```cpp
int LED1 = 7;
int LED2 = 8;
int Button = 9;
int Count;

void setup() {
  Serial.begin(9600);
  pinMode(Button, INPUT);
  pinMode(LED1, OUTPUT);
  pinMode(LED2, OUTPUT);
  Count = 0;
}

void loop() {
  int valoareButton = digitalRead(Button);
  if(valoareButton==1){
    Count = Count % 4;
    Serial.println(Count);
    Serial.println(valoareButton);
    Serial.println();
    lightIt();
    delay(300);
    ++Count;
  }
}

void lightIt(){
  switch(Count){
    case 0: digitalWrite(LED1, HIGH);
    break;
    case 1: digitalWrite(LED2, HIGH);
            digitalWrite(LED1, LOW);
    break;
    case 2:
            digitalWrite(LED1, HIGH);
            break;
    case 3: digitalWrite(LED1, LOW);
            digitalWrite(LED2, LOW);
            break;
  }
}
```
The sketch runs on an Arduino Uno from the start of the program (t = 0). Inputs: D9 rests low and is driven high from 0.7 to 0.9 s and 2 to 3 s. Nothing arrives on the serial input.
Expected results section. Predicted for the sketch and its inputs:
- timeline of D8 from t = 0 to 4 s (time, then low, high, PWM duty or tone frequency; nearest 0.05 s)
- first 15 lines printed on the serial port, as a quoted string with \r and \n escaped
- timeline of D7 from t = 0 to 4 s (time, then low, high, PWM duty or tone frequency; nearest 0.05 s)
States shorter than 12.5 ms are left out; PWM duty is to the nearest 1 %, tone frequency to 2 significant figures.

0 s low; 2 s high; 2.6 s low
"0\r\n1\r\n\r\n1\r\n1\r\n\r\n2\r\n1\r\n\r\n3\r\n1\r\n\r\n0\r\n1\r\n\r\n"
0 s low; 0.7 s high; 2 s low; 2.3 s high; 2.6 s low; 2.9 s high
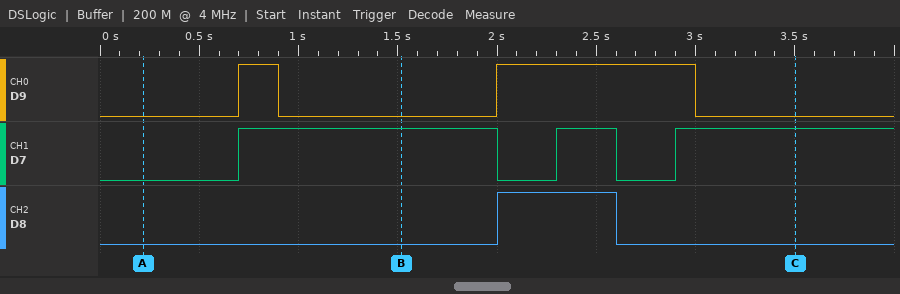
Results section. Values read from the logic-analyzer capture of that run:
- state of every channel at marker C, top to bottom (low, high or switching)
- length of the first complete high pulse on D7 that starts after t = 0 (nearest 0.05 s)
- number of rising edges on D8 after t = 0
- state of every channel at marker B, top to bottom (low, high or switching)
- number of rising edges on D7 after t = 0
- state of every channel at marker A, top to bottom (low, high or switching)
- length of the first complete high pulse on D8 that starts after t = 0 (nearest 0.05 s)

D9 low, D7 high, D8 low
1.30 s
1
D9 low, D7 high, D8 low
3
D9 low, D7 low, D8 low
0.60 s
